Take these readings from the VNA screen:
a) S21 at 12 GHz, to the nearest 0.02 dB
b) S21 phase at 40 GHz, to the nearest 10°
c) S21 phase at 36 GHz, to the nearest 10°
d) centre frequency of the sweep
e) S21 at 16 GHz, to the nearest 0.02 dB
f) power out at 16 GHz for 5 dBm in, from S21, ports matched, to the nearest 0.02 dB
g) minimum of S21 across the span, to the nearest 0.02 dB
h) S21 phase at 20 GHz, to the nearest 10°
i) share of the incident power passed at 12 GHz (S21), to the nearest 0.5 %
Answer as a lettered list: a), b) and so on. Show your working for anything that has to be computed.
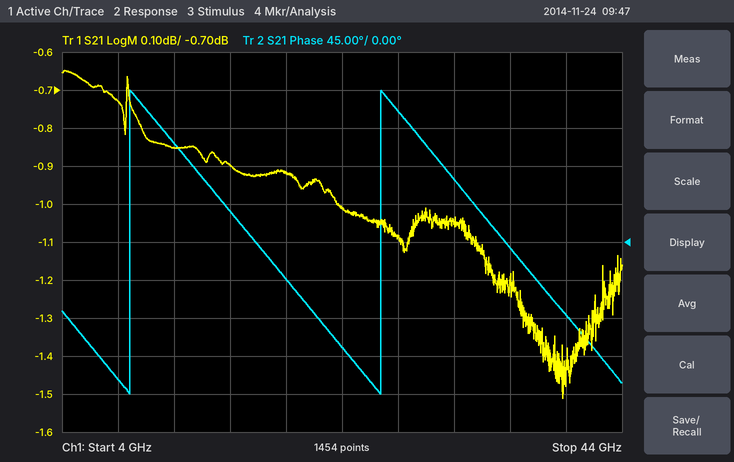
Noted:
a) -0.86 dB
b) -90°
c) -10°
d) 24 GHz
e) -0.90 dB
f) 5 dBm + (-0.90 dB) = 4.10 dBm
g) -1.52 dB
h) -40°
i) 10^(-0.86/10) ≈ 82.0 %
